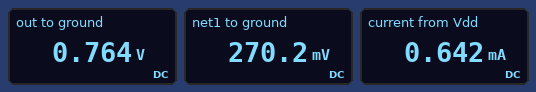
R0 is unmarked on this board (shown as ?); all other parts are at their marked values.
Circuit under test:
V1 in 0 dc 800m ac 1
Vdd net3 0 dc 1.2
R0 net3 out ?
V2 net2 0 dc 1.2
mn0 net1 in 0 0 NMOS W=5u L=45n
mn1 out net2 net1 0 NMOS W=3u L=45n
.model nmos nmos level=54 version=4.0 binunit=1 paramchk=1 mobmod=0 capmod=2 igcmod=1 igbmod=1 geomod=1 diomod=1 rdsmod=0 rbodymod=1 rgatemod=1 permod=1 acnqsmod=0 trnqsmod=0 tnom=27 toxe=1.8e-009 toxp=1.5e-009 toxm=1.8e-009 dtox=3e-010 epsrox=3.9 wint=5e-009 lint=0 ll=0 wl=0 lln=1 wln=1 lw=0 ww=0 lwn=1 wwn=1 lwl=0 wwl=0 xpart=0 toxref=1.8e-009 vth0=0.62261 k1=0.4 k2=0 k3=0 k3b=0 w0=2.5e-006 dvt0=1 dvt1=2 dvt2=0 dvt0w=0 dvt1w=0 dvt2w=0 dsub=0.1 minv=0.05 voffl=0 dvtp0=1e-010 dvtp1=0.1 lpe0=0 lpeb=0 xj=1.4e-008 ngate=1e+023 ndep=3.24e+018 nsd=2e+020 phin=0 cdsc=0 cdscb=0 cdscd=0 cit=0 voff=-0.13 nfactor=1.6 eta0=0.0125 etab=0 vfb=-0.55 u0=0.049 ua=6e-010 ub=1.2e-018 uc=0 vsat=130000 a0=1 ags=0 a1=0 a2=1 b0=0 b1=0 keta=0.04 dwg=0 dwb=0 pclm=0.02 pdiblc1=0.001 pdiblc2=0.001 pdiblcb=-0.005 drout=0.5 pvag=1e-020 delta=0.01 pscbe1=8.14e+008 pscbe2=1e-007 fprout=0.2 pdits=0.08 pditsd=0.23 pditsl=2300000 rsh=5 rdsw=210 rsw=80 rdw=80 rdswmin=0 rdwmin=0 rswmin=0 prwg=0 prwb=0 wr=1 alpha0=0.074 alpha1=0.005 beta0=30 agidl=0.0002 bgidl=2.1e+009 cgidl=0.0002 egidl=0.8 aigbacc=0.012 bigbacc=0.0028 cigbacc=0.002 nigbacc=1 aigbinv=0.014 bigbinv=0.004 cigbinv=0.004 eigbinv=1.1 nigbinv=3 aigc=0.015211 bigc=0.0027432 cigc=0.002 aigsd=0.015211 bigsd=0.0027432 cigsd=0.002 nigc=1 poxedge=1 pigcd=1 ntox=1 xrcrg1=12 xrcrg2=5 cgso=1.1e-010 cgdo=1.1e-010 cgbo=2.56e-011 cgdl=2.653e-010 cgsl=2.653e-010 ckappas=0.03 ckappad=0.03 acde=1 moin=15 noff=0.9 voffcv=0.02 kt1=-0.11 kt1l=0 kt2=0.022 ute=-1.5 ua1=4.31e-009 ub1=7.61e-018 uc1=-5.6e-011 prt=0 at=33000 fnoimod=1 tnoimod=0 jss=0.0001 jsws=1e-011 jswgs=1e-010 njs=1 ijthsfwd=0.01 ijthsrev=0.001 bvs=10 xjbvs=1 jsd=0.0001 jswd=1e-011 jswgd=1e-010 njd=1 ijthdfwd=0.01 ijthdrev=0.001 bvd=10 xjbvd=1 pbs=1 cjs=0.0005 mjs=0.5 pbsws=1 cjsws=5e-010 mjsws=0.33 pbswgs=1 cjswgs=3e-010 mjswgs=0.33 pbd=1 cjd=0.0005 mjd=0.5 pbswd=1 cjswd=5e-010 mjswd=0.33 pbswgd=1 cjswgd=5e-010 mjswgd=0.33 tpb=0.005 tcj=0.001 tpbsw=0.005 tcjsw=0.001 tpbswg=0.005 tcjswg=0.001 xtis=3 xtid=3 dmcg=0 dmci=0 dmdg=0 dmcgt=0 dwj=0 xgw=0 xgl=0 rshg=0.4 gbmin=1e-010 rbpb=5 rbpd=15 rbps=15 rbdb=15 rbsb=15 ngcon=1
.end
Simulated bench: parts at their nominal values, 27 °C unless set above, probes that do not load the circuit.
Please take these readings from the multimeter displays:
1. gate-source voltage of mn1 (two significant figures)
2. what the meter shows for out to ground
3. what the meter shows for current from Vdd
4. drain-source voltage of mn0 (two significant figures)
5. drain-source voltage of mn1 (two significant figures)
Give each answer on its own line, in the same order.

930 mV
0.764 V
0.642 mA
270 mV
490 mV
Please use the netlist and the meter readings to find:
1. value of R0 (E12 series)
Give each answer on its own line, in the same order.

680 Ω
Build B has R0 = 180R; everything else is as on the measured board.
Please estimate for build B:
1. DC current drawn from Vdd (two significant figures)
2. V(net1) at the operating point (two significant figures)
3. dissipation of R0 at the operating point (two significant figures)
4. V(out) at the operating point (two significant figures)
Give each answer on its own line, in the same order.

650 µA
290 mV
76 µW
1.1 V
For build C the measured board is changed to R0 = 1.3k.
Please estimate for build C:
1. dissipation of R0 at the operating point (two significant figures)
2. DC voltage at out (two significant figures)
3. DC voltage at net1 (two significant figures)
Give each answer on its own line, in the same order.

490 µW
400 mV
220 mV
